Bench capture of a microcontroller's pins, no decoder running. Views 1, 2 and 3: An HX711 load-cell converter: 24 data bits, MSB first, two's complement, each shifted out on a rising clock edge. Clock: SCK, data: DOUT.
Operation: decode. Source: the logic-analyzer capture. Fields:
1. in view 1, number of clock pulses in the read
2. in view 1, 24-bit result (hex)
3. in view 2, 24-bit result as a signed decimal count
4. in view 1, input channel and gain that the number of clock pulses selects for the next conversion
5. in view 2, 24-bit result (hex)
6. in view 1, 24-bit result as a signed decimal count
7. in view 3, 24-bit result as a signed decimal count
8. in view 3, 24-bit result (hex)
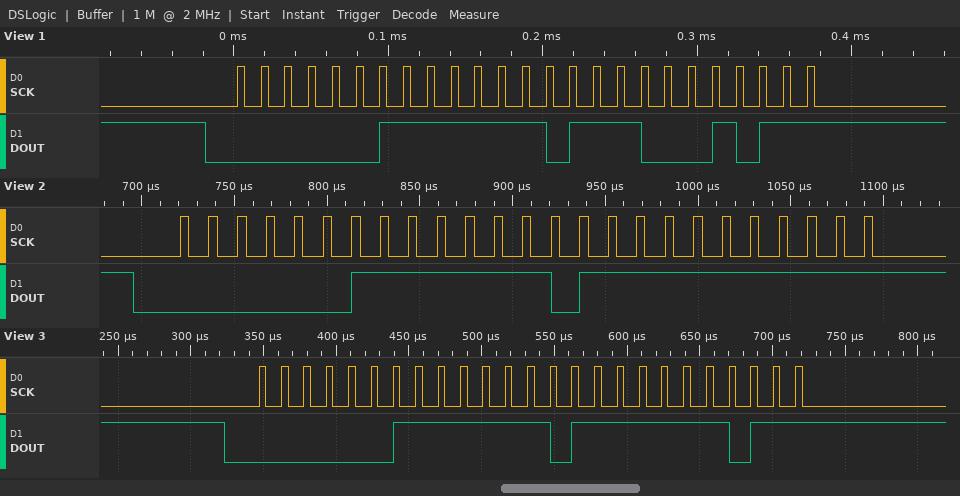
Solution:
25
0x03FB8B
261119
channel A, gain 128
0x03FBFF
261003
261115
0x03FBFB
